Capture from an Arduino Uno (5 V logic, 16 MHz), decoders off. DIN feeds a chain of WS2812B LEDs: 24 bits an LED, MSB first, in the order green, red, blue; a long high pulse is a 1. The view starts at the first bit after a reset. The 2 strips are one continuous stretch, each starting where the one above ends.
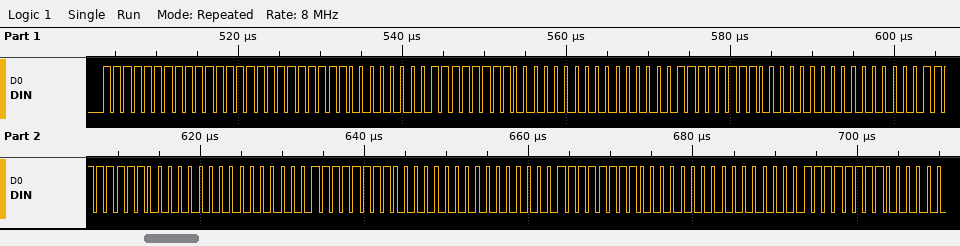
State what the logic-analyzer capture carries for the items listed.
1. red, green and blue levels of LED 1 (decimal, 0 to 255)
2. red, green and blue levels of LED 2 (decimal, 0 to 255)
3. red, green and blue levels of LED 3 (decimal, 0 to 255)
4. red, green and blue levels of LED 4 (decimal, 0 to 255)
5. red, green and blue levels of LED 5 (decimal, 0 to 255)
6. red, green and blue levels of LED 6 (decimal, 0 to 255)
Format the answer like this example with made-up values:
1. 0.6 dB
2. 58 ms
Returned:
1. 255, 255, 255
2. 255, 0, 0
3. 255, 0, 0
4. 255, 0, 0
5. 255, 0, 0
6. 255, 0, 0
